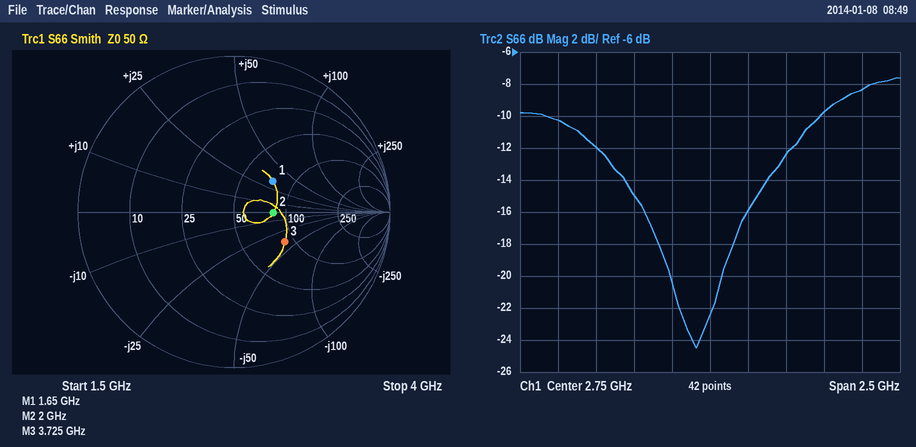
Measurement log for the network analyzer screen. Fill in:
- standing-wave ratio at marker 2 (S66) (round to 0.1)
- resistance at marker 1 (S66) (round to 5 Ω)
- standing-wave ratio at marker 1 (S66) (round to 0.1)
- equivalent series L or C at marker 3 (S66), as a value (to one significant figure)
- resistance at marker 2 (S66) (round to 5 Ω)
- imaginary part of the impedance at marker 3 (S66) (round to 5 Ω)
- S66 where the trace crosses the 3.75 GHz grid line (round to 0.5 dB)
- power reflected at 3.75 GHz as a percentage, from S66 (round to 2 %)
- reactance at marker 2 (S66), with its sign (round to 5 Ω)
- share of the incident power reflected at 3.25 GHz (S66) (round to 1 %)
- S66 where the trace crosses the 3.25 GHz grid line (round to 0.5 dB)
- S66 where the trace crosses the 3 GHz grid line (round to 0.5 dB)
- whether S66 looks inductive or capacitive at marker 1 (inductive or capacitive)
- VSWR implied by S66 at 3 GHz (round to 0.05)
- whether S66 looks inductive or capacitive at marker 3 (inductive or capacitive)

1.7
75 Ω
1.9
1 pF
85 Ω
-40 Ω
-8.5 dB
14 %
0 Ω
6 %
-12.5 dB
-16.0 dB
inductive
1.40
capacitive
